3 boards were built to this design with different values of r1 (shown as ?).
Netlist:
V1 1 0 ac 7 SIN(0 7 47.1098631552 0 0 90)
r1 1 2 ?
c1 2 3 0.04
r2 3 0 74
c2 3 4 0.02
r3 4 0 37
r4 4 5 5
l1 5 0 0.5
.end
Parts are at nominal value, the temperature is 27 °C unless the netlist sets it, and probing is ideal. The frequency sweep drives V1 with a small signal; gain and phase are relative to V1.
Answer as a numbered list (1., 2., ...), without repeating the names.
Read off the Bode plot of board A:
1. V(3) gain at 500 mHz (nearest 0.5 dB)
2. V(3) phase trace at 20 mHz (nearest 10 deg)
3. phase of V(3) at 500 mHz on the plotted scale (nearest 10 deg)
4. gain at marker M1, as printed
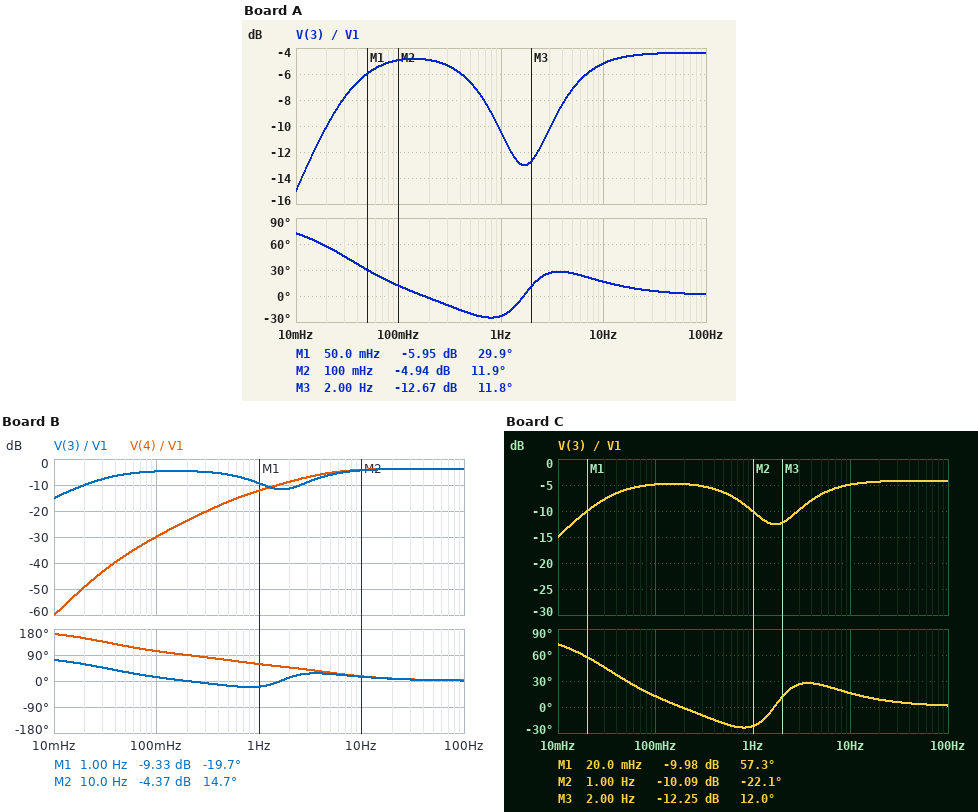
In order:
1. -6.5 dB
2. 60 deg
3. -20 deg
4. -5.95 dB
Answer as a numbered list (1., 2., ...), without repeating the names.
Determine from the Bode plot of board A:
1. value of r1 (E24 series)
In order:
1. 16 Ω
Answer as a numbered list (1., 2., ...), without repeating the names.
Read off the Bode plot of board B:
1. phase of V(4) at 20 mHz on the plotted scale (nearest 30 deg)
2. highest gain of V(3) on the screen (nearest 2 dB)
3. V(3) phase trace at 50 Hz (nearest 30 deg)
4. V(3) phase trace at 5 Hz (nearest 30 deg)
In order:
1. 150 deg
2. -4 dB
3. 0 deg
4. 30 deg
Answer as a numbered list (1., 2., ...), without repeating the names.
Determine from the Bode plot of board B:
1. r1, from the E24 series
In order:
1. 13 Ω
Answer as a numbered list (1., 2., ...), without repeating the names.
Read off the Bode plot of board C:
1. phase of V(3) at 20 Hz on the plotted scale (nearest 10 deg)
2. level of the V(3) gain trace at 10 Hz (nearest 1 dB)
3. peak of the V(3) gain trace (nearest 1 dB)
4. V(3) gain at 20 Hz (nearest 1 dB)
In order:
1. 10 deg
2. -5 dB
3. -4 dB
4. -4 dB
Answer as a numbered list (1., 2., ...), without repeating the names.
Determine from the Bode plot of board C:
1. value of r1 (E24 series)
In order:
1. 15 Ω
